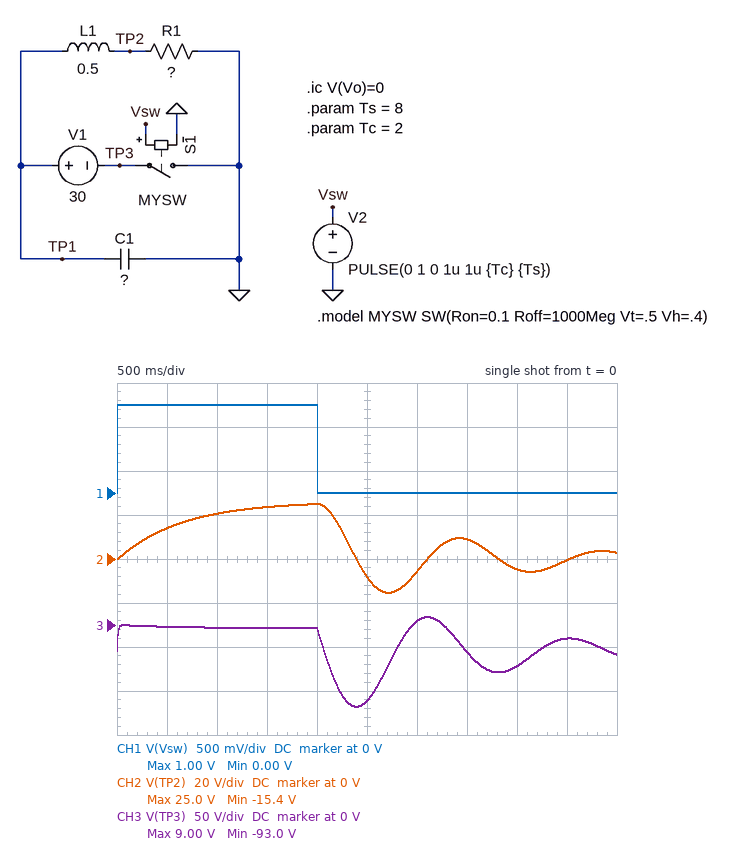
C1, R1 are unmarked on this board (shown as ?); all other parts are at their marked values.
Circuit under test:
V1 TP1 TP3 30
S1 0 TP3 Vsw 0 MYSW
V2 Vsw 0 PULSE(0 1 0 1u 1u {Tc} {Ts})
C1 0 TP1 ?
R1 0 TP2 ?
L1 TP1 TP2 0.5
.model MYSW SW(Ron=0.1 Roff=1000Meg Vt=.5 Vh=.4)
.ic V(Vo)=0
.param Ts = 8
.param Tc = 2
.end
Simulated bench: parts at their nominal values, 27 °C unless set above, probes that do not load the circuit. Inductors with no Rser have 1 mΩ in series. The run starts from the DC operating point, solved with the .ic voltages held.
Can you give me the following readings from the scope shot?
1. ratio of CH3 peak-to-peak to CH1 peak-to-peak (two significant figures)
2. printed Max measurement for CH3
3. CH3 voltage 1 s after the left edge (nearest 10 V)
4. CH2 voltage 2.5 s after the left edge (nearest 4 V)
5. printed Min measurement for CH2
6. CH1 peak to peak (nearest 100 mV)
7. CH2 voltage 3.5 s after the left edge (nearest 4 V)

100
9.00 V
0 V
-8 V
-15.4 V
1.0 V
8 V
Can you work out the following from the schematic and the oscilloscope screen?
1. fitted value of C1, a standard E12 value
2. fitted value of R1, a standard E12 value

100 mF
0.68 Ω
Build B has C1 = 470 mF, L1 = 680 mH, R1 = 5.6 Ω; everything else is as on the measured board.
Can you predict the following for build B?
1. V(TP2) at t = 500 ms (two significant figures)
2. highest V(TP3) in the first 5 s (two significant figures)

29 V
-470 mV
